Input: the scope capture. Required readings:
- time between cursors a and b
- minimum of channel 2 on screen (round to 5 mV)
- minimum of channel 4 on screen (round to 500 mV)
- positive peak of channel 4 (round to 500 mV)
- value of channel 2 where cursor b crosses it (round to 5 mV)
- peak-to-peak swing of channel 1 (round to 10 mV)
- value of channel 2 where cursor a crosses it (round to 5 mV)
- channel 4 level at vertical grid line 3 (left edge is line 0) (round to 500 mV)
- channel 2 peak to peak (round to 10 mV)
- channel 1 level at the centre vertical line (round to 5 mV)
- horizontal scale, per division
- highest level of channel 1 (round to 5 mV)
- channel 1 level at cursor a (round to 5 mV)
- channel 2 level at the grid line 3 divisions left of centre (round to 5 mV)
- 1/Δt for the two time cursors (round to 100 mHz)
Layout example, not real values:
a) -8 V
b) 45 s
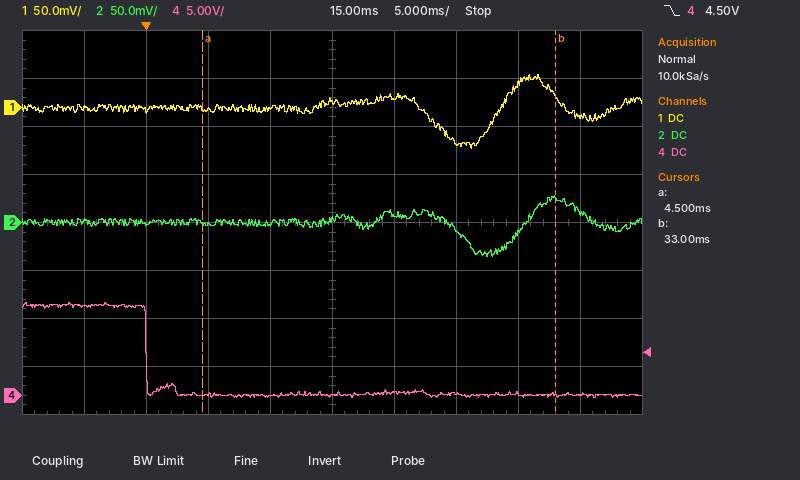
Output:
a) 28.5 ms
b) -35 mV
c) 0.0 V
d) 9.5 V
e) 25 mV
f) 80 mV
g) 0 mV
h) 0.0 V
i) 60 mV
j) 5 mV
k) 5 ms
l) 35 mV
m) 0 mV
n) 0 mV
o) 35.1 Hz
